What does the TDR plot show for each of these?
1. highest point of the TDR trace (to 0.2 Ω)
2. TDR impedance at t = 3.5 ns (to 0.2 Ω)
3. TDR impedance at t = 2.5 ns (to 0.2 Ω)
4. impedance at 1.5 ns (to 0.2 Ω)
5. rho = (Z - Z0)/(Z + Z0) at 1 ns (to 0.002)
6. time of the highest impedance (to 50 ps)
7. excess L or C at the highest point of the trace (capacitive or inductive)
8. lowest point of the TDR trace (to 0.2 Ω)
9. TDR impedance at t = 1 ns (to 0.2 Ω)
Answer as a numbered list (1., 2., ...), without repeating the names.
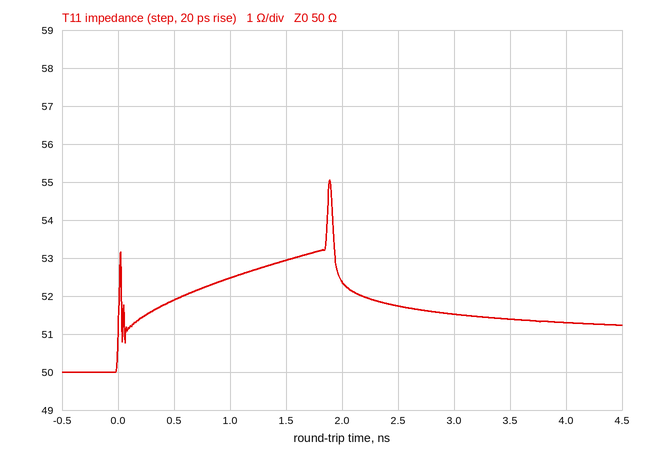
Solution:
1. 55.0 Ω
2. 51.4 Ω
3. 51.8 Ω
4. 53.0 Ω
5. +0.024
6. 1.90 ns
7. inductive
8. 50.0 Ω
9. 52.4 Ω
